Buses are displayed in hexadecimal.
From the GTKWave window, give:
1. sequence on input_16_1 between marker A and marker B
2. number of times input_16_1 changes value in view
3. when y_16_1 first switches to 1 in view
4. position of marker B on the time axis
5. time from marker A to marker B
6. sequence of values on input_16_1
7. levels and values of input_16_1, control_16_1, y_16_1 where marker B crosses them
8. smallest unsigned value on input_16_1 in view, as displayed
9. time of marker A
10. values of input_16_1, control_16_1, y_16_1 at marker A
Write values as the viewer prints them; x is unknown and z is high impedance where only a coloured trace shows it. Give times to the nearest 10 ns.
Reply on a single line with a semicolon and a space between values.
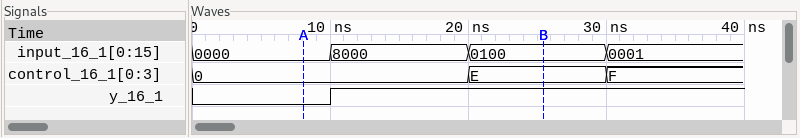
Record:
0000, 8000, 0100; 3; 10 ns; 30 ns; 20 ns; 0000, 8000, 0100, 0001; input_16_1=0100, control_16_1=E, y_16_1=1; 0000; 10 ns; input_16_1=0000, control_16_1=0, y_16_1=0
